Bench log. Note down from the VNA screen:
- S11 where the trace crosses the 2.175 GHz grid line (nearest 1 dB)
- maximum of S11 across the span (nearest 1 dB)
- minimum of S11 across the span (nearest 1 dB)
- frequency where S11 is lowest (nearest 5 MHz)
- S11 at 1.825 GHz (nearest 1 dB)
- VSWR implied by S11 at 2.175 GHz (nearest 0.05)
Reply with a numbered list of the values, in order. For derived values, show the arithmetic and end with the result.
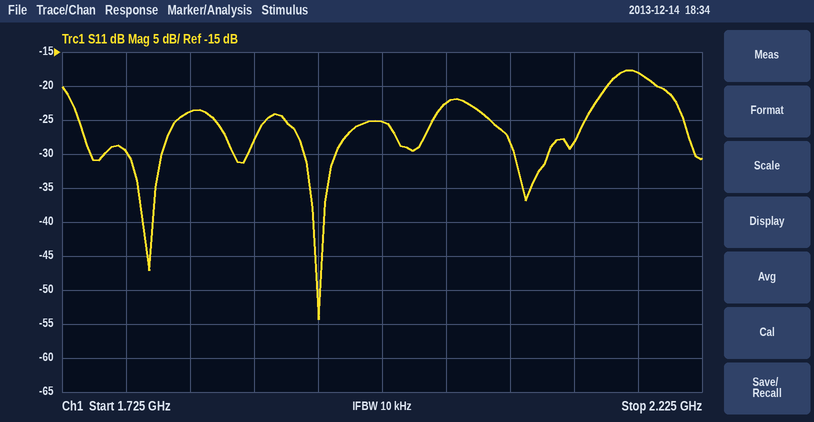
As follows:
1. -18 dB
2. -18 dB
3. -54 dB
4. 1.925 GHz
5. -24 dB
6. |Γ| = 10^(-18/20) = 0.1259; VSWR = (1 + 0.1259)/(1 − 0.1259) ≈ 1.29, so 1.30 to the nearest 0.05
